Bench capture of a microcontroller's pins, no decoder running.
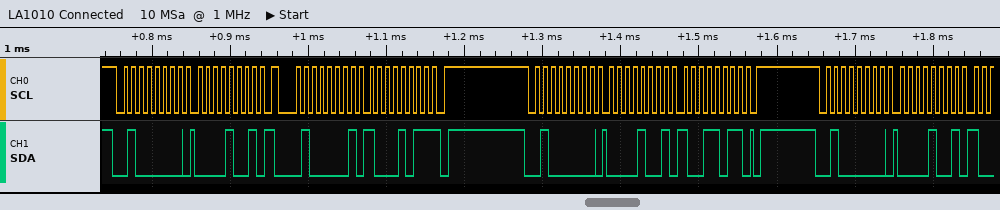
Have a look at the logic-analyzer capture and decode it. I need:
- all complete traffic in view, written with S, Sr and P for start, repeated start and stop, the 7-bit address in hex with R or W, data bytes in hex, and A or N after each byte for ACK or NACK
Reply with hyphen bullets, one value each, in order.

- S 20W A 09 A Sr 20R A 8B N P S 20W A 09 A 9B A P S 20W A 09 A
